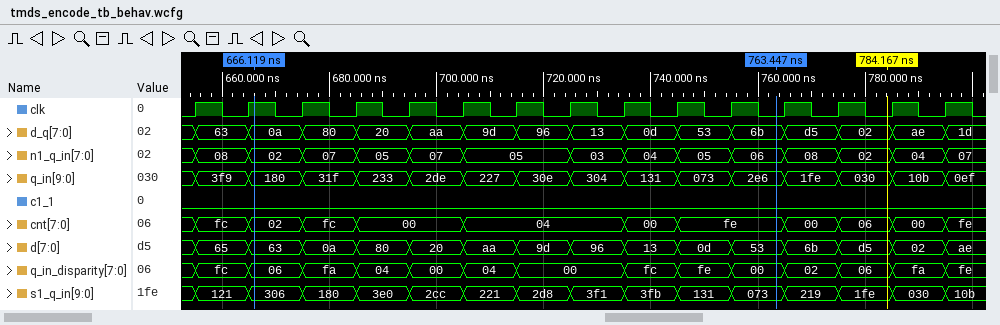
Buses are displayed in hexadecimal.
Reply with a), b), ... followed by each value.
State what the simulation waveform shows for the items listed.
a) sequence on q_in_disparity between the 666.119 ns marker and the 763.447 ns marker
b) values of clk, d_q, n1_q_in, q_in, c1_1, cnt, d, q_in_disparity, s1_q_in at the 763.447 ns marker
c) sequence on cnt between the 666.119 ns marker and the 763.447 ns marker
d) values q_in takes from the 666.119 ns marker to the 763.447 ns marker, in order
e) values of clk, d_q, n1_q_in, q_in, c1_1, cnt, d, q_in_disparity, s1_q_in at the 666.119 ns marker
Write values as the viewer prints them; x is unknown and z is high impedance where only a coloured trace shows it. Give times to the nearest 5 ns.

a) 06, fa, 04, 00, 04, 00, fc, fe, 00
b) clk=0, d_q=6b, n1_q_in=06, q_in=2e6, c1_1=0, cnt=fe, d=53, q_in_disparity=00, s1_q_in=073
c) 02, fc, 00, 04, 00, fe
d) 180, 31f, 233, 2de, 227, 30e, 304, 131, 073, 2e6
e) clk=1, d_q=0a, n1_q_in=02, q_in=180, c1_1=0, cnt=02, d=63, q_in_disparity=06, s1_q_in=306
